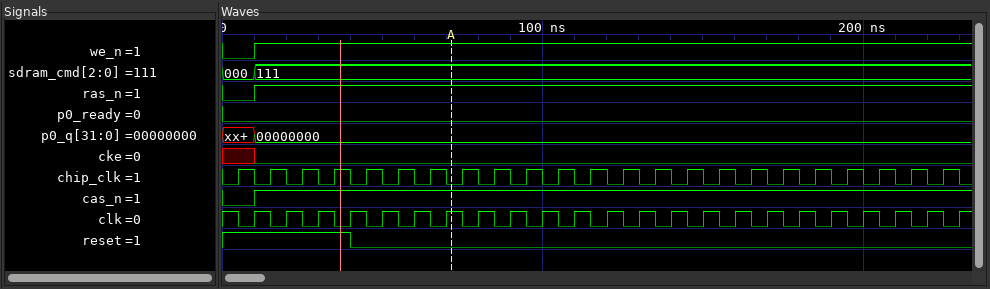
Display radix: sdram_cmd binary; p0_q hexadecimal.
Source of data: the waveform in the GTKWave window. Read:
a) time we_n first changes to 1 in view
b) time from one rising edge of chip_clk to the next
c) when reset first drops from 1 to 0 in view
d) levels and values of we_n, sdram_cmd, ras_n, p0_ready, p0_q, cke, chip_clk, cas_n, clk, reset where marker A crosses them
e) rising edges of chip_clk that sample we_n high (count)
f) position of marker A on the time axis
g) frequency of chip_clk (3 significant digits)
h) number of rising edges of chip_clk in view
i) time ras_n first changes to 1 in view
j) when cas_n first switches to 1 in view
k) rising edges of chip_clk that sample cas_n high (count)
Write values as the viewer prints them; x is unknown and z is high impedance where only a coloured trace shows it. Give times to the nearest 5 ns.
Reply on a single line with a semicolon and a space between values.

10 ns; 10 ns; 40 ns; we_n=1, sdram_cmd=111, ras_n=1, p0_ready=0, p0_q=00000000, cke=0, chip_clk=0, cas_n=1, clk=1, reset=0; 22; 70 ns; 100 MHz; 23; 10 ns; 10 ns; 22
